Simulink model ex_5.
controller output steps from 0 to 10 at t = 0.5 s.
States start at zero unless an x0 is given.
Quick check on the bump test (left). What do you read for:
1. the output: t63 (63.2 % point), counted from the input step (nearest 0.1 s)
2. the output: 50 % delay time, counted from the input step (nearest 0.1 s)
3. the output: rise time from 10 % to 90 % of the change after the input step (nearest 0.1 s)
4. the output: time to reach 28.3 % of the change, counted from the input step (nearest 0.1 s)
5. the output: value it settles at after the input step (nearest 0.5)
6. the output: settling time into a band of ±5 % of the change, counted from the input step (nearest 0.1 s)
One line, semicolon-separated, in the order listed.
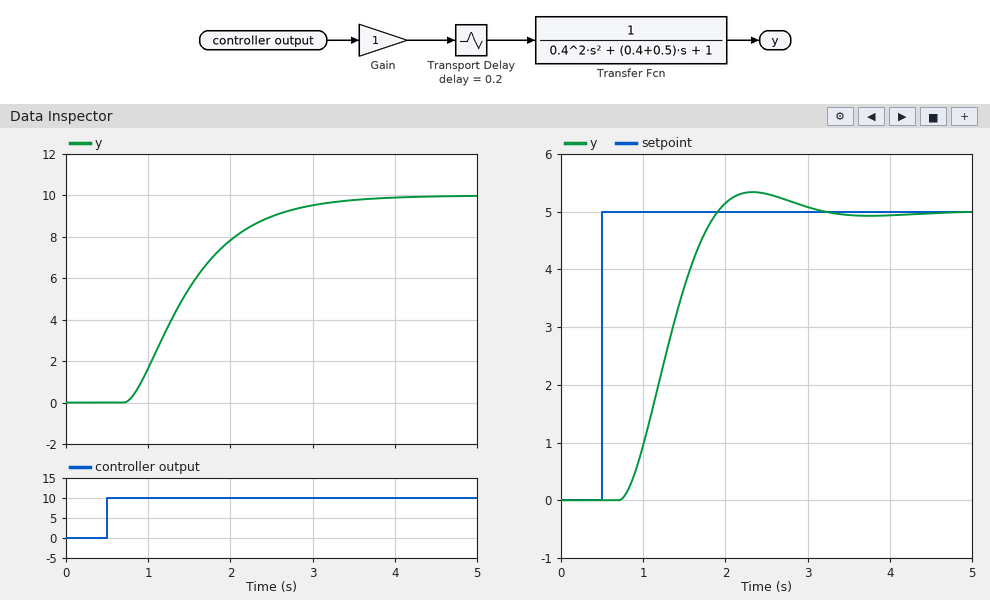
1.1 s; 0.9 s; 1.6 s; 0.6 s; 10.0; 2.5 s
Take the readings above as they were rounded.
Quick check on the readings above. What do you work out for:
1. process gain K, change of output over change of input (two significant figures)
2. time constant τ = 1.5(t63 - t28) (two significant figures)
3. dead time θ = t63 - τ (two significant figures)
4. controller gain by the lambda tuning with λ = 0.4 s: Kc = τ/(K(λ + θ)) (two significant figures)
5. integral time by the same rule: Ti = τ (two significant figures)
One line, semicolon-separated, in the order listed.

1.0; 0.75 s; 0.35 s; 1.0; 0.75 s
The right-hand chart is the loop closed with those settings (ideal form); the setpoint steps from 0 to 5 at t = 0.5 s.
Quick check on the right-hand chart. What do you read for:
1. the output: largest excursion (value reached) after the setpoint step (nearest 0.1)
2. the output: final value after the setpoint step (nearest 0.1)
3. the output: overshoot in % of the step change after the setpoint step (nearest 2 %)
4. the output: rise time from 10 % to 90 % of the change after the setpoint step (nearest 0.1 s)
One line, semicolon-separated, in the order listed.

5.3; 5.0; 6 %; 0.8 s
